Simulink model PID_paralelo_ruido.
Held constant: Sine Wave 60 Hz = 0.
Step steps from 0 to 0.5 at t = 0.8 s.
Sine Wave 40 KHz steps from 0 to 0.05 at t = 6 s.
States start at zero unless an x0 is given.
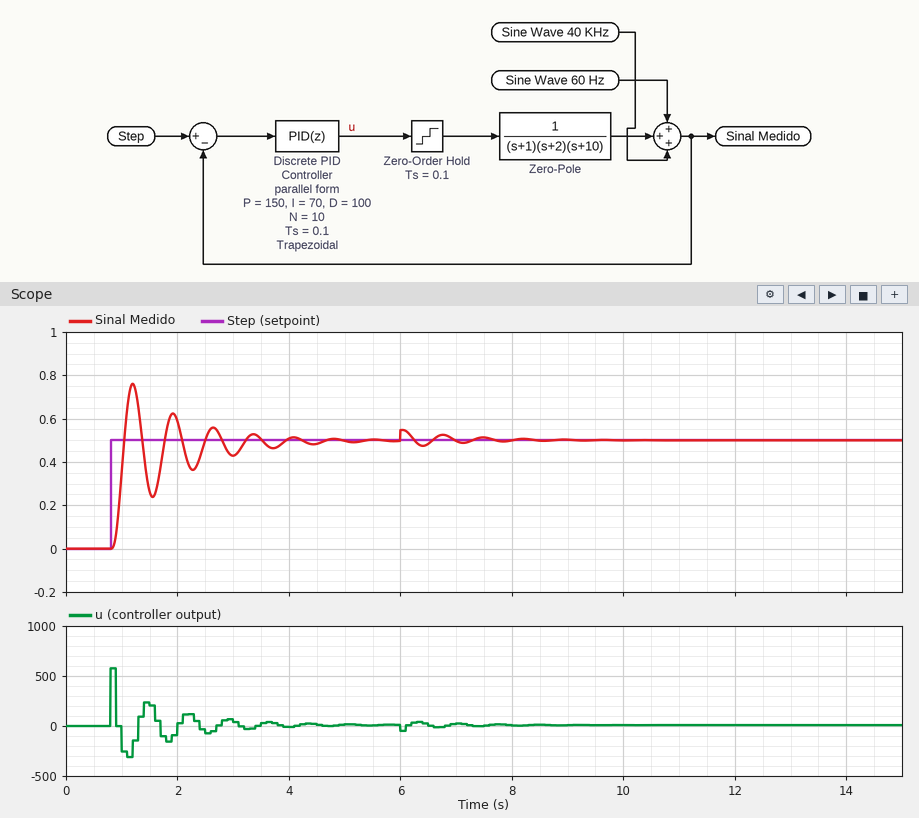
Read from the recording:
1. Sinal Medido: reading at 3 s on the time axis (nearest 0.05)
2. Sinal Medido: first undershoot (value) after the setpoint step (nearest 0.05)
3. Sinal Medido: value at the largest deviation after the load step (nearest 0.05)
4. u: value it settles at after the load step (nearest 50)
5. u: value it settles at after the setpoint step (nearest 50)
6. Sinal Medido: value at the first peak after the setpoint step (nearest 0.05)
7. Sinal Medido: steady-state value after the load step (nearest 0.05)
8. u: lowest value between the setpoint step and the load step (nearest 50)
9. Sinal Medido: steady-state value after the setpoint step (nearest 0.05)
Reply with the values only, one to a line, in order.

0.45
0.25
0.55
0
0
0.75
0.50
-300
0.50
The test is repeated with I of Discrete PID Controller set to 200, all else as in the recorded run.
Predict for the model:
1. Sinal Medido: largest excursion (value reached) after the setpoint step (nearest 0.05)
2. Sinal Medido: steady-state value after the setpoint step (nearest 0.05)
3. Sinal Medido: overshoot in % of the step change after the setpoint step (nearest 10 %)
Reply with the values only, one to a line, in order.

0.80
0.50
60 %
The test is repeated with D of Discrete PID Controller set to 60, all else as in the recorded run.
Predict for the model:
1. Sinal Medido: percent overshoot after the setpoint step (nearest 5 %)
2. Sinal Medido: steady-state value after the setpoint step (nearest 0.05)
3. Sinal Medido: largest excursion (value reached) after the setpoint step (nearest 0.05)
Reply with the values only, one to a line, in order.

35 %
0.50
0.65
